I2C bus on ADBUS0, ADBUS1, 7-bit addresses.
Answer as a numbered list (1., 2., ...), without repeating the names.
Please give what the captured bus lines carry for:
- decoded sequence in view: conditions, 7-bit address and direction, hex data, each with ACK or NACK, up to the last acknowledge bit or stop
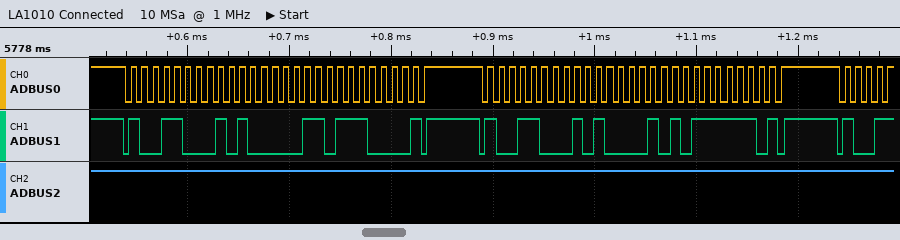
1. start, address 4C write NACK, 41 NACK, 70 NACK, stop, start, address 4C write NACK, 42 NACK, 7E NACK, stop
